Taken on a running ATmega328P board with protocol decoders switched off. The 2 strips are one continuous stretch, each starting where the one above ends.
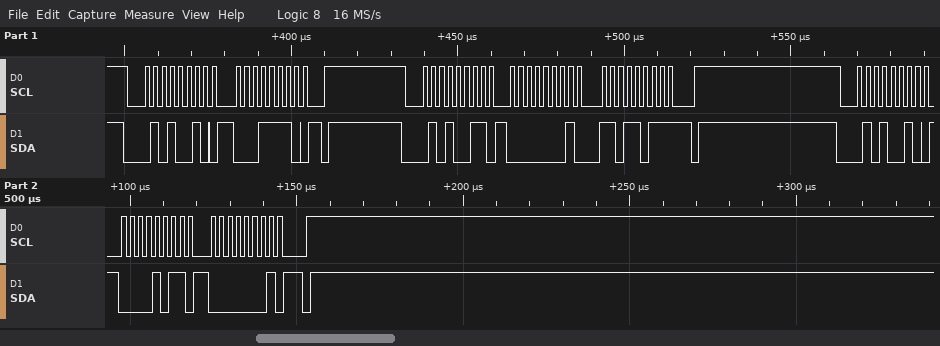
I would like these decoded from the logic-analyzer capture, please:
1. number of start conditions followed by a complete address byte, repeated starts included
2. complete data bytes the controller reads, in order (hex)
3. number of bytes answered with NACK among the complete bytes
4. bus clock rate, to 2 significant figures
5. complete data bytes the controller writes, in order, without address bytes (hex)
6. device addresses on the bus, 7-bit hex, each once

3
01 DB
1
400 kHz
1E 0B 01
0x29
